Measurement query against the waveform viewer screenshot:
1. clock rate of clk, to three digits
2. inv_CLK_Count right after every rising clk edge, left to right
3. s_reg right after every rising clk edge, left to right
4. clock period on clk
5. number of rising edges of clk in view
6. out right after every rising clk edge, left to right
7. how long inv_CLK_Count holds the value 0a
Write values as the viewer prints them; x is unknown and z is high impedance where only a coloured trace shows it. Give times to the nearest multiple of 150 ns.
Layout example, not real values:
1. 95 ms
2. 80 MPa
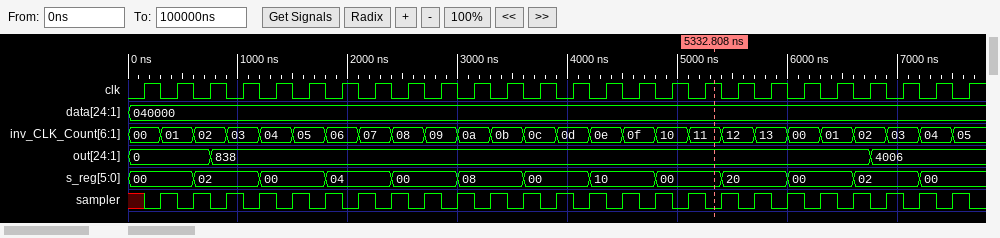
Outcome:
1. 3.33 MHz
2. 00, 01, 02, 03, 04, 05, 06, 07, 08, 09, 0a, 0b, 0c, 0d, 0e, 0f, 10, 11, 12, 13, 00, 01, 02, 03, 04, 05
3. 00, 00, 02, 02, 00, 00, 04, 04, 00, 00, 08, 08, 00, 00, 10, 10, 00, 00, 20, 20, 00, 00, 02, 02, 00, 00
4. 300 ns
5. 26
6. 0, 0, 838, 838, 838, 838, 838, 838, 838, 838, 838, 838, 838, 838, 838, 838, 838, 838, 838, 838, 838, 838, 4006, 4006, 4006, 4006
7. 300 ns
